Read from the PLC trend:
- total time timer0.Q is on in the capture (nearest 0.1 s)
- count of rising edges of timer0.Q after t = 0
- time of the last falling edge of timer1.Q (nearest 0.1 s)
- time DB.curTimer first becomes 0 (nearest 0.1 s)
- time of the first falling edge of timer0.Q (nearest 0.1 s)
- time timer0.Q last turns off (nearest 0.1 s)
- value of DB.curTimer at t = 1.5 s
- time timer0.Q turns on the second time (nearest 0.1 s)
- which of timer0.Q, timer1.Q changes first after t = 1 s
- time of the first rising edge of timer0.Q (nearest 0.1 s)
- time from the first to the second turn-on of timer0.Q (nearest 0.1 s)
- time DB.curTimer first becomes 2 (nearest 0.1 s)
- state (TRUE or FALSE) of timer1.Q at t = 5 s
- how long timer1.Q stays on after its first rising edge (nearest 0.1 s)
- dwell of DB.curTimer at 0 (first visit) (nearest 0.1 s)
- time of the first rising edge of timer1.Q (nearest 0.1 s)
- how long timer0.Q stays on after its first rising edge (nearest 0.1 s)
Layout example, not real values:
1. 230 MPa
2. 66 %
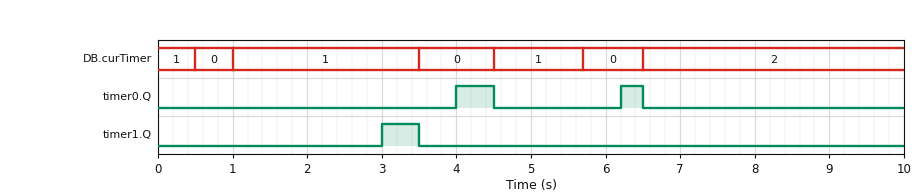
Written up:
1. 0.8 s
2. 2
3. 3.5 s
4. 0.5 s
5. 4.5 s
6. 6.5 s
7. 1
8. 6.2 s
9. timer1.Q
10. 4.0 s
11. 2.2 s
12. 6.5 s
13. FALSE
14. 0.5 s
15. 0.5 s
16. 3.0 s
17. 0.5 s
